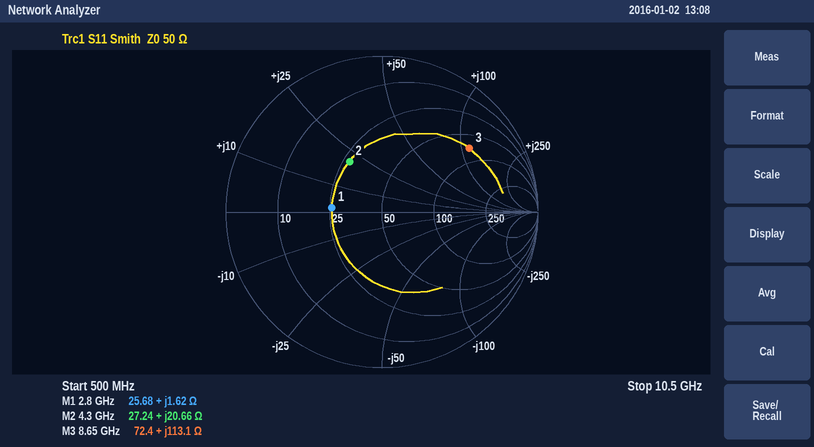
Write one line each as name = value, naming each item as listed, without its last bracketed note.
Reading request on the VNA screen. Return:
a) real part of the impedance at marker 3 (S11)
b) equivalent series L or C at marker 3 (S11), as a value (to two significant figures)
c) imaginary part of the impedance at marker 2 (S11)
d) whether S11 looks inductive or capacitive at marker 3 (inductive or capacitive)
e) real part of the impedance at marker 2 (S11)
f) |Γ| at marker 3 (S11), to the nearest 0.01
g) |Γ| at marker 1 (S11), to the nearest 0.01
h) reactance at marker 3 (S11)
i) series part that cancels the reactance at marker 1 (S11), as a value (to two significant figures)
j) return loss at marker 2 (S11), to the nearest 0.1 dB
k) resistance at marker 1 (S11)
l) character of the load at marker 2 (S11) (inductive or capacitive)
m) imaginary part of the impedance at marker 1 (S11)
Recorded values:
real part of the impedance at marker 3 = 72.4 Ω
equivalent series L or C at marker 3 (S11), as a value = 2.1 nH
imaginary part of the impedance at marker 2 = +20.66 Ω
whether S11 looks inductive or capacitive at marker 3 = inductive
real part of the impedance at marker 2 = 27.24 Ω
|Γ| at marker 3 (S11), to the nearest 0.01 = 0.69
|Γ| at marker 1 (S11), to the nearest 0.01 = 0.32
reactance at marker 3 = +113.1 Ω
series part that cancels the reactance at marker 1 (S11), as a value = 35 pF
return loss at marker 2 (S11), to the nearest 0.1 dB = 8.3 dB
resistance at marker 1 = 25.68 Ω
character of the load at marker 2 (S11) = inductive
imaginary part of the impedance at marker 1 = +1.62 Ω
